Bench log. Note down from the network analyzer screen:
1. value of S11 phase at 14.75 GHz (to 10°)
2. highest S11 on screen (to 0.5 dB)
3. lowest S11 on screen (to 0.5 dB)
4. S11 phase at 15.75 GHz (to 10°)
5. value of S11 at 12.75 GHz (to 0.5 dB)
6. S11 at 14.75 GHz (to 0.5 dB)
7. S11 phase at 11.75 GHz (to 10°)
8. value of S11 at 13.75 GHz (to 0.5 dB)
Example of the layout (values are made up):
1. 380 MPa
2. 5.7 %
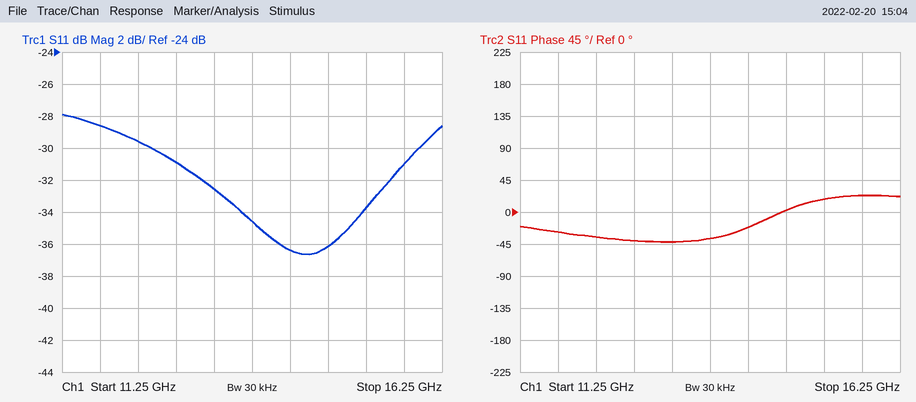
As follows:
1. 0°
2. -28.0 dB
3. -36.5 dB
4. 20°
5. -31.0 dB
6. -36.0 dB
7. -30°
8. -34.5 dB
